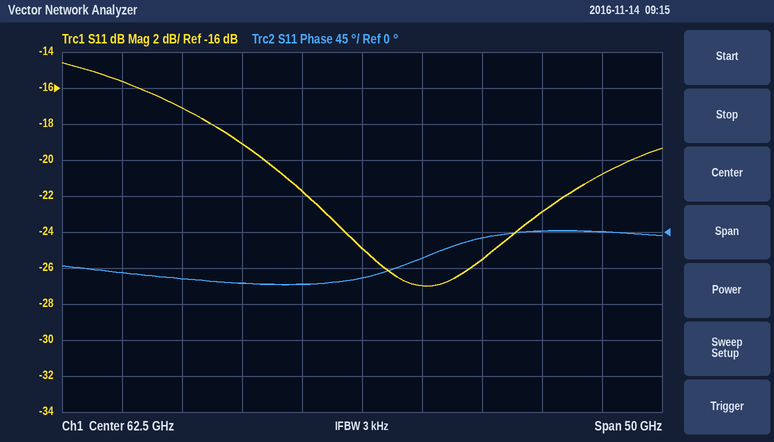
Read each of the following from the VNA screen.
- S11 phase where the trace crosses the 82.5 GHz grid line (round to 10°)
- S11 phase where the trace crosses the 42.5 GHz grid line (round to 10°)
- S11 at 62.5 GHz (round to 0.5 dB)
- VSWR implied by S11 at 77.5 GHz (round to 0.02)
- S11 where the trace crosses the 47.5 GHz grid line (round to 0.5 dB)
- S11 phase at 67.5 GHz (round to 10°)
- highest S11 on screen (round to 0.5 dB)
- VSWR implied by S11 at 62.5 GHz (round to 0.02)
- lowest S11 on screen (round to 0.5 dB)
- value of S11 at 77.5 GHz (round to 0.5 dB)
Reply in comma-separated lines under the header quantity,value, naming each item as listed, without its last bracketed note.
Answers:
quantity,value
S11 phase where the trace crosses the 82.5 GHz grid line,0°
S11 phase where the trace crosses the 42.5 GHz grid line,-50°
S11 at 62.5 GHz,-25.0 dB
VSWR implied by S11 at 77.5 GHz,1.16
S11 where the trace crosses the 47.5 GHz grid line,-17.0 dB
S11 phase at 67.5 GHz,-30°
highest S11 on screen,-14.5 dB
VSWR implied by S11 at 62.5 GHz,1.12
lowest S11 on screen,-27.0 dB
value of S11 at 77.5 GHz,-23.0 dB
